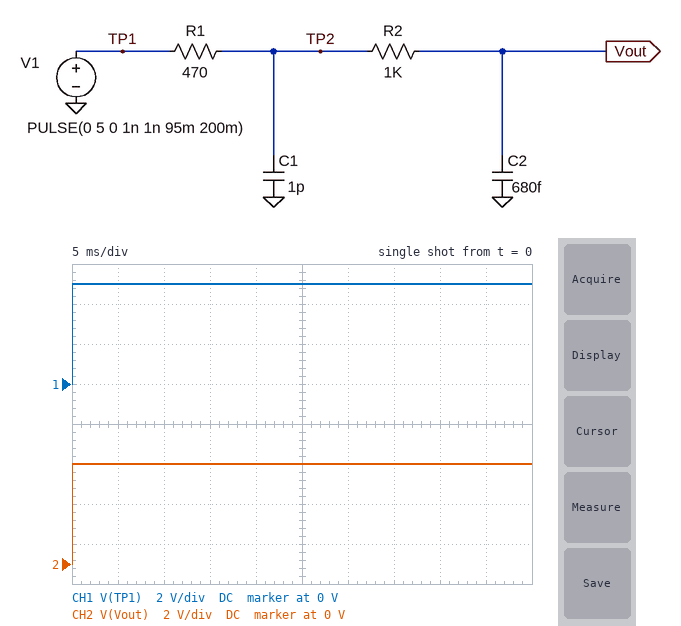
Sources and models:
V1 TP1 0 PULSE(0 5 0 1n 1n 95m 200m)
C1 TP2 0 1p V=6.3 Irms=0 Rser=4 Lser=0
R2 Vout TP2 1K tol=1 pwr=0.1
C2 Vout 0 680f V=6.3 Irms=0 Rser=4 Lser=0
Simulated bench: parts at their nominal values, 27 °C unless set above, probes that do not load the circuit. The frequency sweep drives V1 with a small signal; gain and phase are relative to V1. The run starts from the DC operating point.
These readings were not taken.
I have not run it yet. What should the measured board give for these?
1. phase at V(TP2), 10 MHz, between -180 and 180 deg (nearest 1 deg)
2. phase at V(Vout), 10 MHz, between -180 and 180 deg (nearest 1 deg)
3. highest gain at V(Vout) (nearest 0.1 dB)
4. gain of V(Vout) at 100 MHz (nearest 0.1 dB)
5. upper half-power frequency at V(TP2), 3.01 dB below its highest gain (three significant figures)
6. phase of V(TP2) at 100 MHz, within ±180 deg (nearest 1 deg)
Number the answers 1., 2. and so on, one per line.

1. -3 deg
2. -5 deg
3. 0 dB
4. -2.1 dB
5. 185 MHz
6. -23 deg
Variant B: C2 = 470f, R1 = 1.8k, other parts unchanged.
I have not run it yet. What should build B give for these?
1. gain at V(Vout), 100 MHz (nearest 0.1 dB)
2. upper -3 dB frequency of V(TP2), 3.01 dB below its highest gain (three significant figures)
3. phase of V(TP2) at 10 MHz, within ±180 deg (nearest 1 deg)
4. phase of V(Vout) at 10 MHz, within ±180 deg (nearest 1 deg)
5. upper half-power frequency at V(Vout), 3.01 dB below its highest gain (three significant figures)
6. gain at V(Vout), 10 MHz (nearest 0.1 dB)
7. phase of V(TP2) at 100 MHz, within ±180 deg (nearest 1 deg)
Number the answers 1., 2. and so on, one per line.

1. -6.3 dB
2. 57.4 MHz
3. -9 deg
4. -11 deg
5. 55.8 MHz
6. -0.1 dB
7. -55 deg
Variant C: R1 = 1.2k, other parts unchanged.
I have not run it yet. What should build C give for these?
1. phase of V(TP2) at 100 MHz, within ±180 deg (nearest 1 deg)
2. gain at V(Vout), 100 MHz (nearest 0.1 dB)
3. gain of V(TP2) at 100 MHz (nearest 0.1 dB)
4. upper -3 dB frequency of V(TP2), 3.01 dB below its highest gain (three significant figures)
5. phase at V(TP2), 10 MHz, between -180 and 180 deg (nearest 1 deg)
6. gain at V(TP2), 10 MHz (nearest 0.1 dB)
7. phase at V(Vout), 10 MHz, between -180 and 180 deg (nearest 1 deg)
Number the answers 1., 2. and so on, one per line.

1. -45 deg
2. -5.2 dB
3. -4.5 dB
4. 72.2 MHz
5. -7 deg
6. -0.1 dB
7. -10 deg
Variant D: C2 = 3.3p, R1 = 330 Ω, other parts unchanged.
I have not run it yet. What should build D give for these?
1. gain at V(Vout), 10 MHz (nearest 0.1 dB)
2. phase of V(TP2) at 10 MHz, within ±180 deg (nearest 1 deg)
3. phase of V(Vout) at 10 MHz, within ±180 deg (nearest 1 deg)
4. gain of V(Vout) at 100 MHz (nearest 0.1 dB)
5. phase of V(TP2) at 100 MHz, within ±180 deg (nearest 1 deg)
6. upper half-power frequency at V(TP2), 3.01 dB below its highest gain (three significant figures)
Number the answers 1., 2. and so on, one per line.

1. -0.3 dB
2. -5 deg
3. -17 deg
4. -9.6 dB
5. -15 deg
6. 217 MHz
